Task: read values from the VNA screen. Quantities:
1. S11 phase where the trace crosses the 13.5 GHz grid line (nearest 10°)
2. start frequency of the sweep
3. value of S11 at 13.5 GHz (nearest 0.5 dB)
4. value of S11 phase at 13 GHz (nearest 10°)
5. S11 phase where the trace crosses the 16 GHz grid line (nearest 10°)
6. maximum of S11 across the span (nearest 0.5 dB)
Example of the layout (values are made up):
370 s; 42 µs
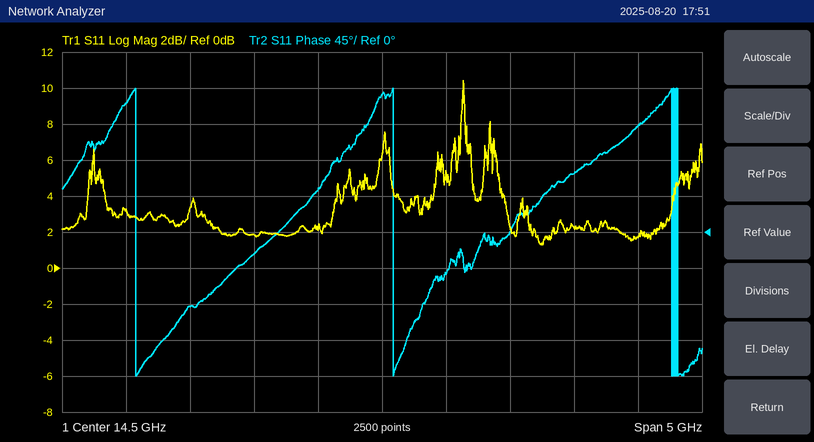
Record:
-30°; 12 GHz; 2.0 dB; -90°; 70°; 10.5 dB
